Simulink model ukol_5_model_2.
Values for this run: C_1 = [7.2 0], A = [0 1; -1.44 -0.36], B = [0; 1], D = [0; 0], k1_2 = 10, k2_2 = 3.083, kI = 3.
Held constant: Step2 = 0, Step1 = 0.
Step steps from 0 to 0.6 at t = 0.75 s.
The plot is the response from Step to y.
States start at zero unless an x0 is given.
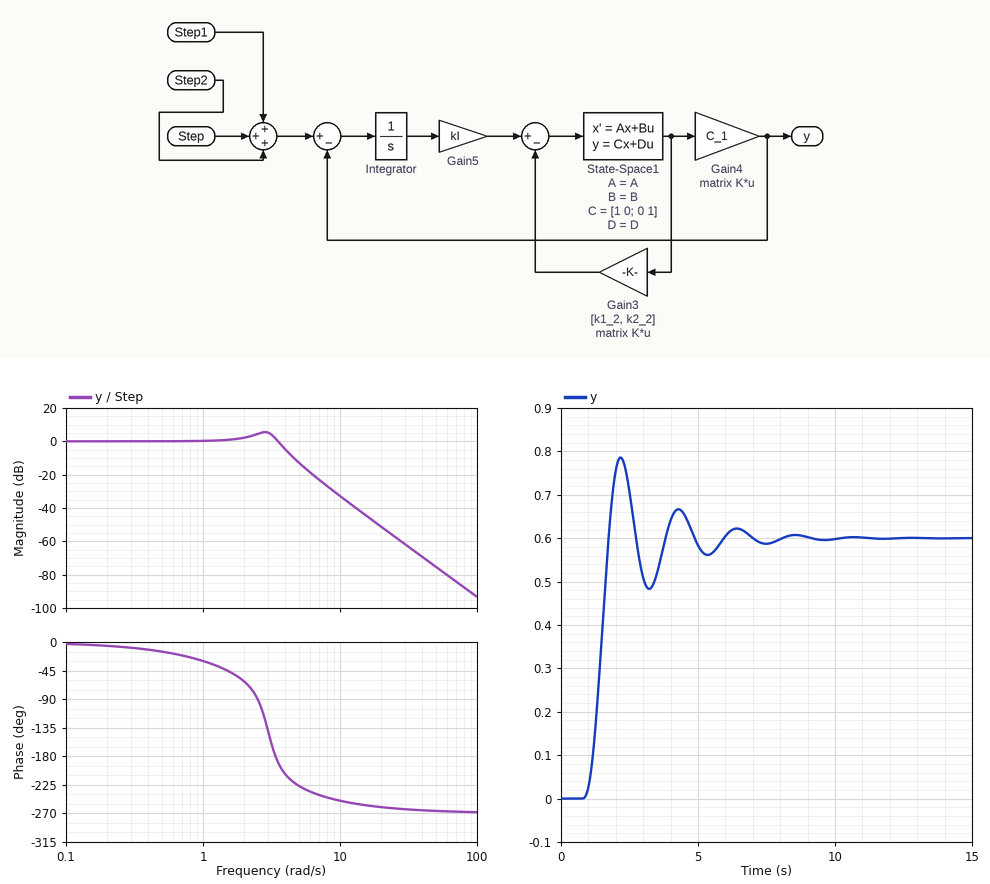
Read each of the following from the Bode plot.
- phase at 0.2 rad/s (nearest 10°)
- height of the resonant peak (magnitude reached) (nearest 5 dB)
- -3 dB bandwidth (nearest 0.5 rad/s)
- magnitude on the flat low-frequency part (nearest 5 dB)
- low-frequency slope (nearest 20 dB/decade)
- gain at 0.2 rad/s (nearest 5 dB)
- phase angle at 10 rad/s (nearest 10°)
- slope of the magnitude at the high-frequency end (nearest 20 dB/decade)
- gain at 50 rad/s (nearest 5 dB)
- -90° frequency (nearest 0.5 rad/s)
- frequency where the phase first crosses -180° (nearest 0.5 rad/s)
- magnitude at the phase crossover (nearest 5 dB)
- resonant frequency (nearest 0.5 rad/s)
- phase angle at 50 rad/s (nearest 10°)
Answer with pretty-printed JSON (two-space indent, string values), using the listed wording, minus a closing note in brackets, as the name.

{
  "phase at 0.2 rad/s": "-10°",
  "height of the resonant peak (magnitude reached)": "5 dB",
  "-3 dB bandwidth": "4.0 rad/s",
  "magnitude on the flat low-frequency part": "0 dB",
  "low-frequency slope": "0 dB/decade",
  "gain at 0.2 rad/s": "0 dB",
  "phase angle at 10 rad/s": "-250°",
  "slope of the magnitude at the high-frequency end": "-60 dB/decade",
  "gain at 50 rad/s": "-75 dB",
  "-90° frequency": "2.5 rad/s",
  "frequency where the phase first crosses -180°": "3.5 rad/s",
  "magnitude at the phase crossover": "0 dB",
  "resonant frequency": "3.0 rad/s",
  "phase angle at 50 rad/s": "-270°"
}
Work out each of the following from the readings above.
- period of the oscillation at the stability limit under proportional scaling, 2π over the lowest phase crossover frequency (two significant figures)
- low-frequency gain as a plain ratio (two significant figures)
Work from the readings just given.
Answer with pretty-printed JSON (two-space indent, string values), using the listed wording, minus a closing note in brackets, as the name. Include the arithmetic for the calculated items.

{
  "period of the oscillation at the stability limit under proportional scaling, 2π over the lowest phase crossover frequency": "2π / 3.5 = 1.8 s",
  "low-frequency gain as a plain ratio": "10^(0 / 20) = 1.0"
}
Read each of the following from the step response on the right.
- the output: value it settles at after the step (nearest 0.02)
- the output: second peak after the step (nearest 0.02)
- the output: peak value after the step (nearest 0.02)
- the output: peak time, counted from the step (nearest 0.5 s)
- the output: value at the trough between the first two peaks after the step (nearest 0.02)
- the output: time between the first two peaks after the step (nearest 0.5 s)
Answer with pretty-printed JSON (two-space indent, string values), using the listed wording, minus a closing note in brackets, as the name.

{
  "the output: value it settles at after the step": "0.60",
  "the output: second peak after the step": "0.66",
  "the output: peak value after the step": "0.78",
  "the output: peak time, counted from the step": "1.5 s",
  "the output: value at the trough between the first two peaks after the step": "0.48",
  "the output: time between the first two peaks after the step": "2.0 s"
}
